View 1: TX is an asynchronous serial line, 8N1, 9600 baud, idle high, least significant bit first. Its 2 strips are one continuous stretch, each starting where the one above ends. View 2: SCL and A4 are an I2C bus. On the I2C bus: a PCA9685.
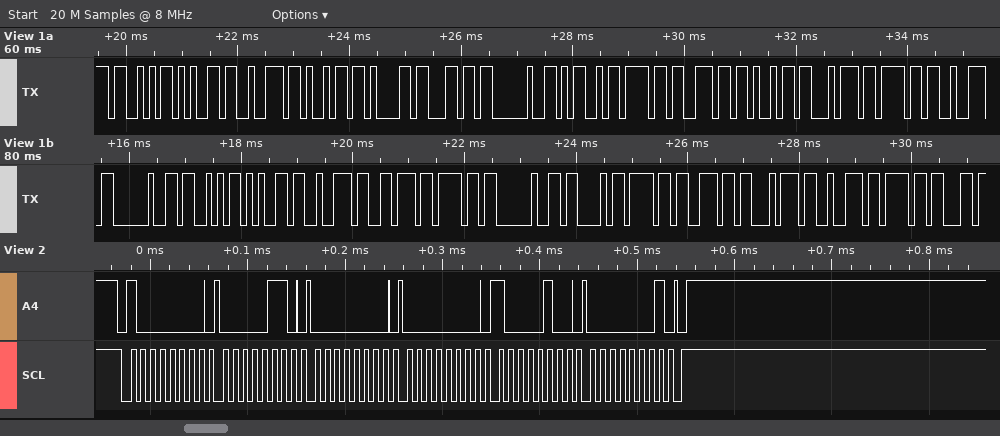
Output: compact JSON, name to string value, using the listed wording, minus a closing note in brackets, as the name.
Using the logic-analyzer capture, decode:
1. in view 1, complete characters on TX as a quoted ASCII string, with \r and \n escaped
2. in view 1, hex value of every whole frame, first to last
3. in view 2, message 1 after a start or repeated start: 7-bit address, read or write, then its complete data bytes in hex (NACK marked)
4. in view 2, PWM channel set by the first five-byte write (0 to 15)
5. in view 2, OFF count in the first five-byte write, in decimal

{"in view 1, complete characters on TX as a quoted ASCII string, with \\r and \\n escaped": "\"Serial Monitor Servo Contro\"", "in view 1, hex value of every whole frame, first to last": "53 65 72 69 61 6C 20 4D 6F 6E 69 74 6F 72 20 53 65 72 76 6F 20 43 6F 6E 74 72 6F", "in view 2, message 1 after a start or repeated start: 7-bit address, read or write, then its complete data bytes in hex": "0x40 write: 06 00 00 84 01", "in view 2, PWM channel set by the first five-byte write": "0", "in view 2, OFF count in the first five-byte write, in decimal": "388"}
